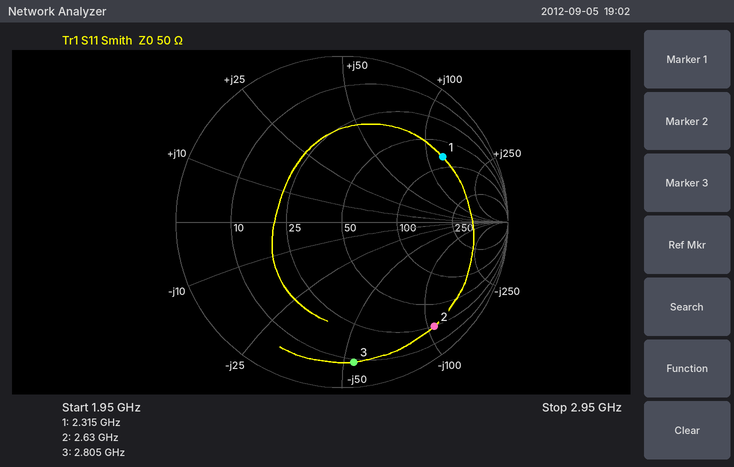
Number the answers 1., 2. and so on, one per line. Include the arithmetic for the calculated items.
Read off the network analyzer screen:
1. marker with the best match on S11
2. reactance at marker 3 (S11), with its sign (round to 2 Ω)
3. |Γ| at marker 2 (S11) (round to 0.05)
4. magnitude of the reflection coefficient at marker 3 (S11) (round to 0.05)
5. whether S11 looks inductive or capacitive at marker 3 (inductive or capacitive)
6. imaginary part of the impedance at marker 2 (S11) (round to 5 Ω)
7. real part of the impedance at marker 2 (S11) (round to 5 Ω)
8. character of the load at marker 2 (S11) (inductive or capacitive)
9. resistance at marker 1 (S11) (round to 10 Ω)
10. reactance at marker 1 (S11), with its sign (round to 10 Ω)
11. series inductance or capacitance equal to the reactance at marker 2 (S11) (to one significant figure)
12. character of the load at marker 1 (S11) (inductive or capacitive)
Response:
1. marker 1
2. -54 Ω
3. 0.85
4. 0.85
5. capacitive
6. -105 Ω
7. 25 Ω
8. capacitive
9. 80 Ω
10. +130 Ω
11. C = 1/(2π × 2.63 GHz × 105 Ω) ≈ 576 fF, so 600 fF to one significant figure
12. inductive
